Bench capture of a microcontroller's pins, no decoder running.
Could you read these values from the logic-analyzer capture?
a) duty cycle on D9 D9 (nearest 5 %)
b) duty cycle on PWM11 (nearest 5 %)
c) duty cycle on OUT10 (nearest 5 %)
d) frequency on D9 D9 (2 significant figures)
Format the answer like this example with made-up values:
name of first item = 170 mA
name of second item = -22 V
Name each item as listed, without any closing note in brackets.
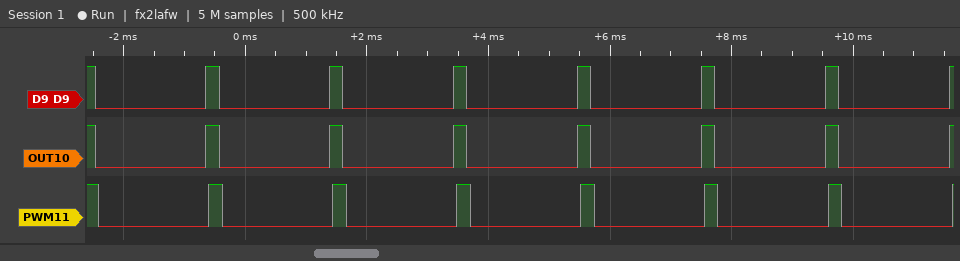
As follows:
duty cycle on D9 D9 = 10 %
duty cycle on PWM11 = 10 %
duty cycle on OUT10 = 10 %
frequency on D9 D9 = 490 Hz
